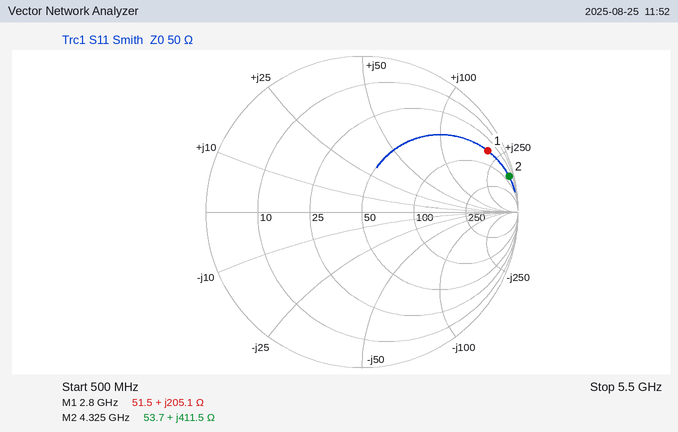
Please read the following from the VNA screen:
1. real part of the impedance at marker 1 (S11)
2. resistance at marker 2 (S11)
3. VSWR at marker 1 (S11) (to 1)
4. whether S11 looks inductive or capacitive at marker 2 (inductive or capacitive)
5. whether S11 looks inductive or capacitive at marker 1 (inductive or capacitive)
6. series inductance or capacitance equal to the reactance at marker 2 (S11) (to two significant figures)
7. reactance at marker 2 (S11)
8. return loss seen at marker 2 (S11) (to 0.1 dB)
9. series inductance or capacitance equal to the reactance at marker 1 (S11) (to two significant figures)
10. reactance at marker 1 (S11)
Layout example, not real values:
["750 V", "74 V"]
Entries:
["51.5 Ω", "53.7 Ω", "18", "inductive", "inductive", "15 nH", "+411.5 Ω", "0.3 dB", "12 nH", "+205.1 Ω"]
